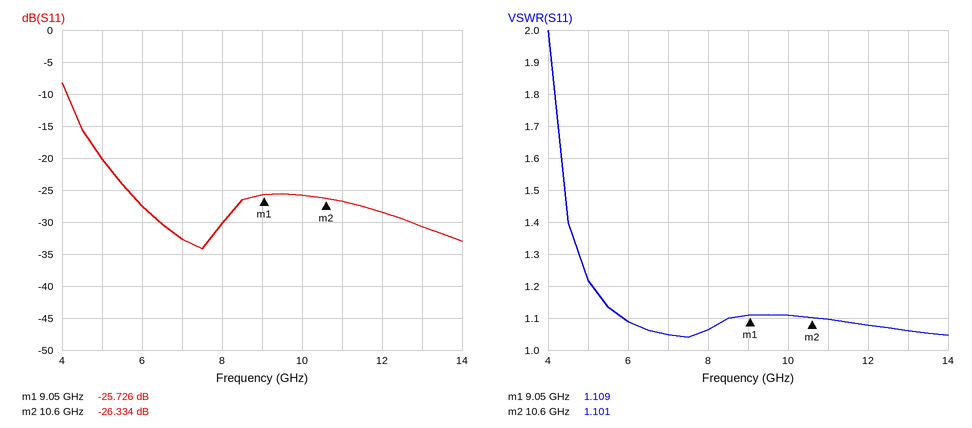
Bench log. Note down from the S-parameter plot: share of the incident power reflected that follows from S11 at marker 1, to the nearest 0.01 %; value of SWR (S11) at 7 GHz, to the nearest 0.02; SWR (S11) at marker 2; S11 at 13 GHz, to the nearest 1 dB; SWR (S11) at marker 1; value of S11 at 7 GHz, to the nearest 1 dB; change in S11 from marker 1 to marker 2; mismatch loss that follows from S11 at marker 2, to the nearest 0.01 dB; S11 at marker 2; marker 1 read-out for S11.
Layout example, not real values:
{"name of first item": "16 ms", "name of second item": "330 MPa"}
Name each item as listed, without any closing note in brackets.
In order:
{"share of the incident power reflected that follows from S11 at marker 1, to the nearest 0.01 %": "0.27 %", "value of SWR (S11) at 7 GHz, to the nearest 0.02": "1.04", "SWR (S11) at marker 2": "1.101", "S11 at 13 GHz, to the nearest 1 dB": "-31 dB", "SWR (S11) at marker 1": "1.109", "value of S11 at 7 GHz, to the nearest 1 dB": "-33 dB", "change in S11 from marker 1 to marker 2": "-0.608 dB", "mismatch loss that follows from S11 at marker 2, to the nearest 0.01 dB": "0.01 dB", "S11 at marker 2": "-26.334 dB", "marker 1 read-out for S11": "-25.726 dB"}
